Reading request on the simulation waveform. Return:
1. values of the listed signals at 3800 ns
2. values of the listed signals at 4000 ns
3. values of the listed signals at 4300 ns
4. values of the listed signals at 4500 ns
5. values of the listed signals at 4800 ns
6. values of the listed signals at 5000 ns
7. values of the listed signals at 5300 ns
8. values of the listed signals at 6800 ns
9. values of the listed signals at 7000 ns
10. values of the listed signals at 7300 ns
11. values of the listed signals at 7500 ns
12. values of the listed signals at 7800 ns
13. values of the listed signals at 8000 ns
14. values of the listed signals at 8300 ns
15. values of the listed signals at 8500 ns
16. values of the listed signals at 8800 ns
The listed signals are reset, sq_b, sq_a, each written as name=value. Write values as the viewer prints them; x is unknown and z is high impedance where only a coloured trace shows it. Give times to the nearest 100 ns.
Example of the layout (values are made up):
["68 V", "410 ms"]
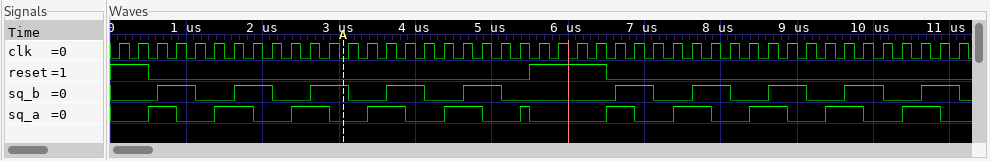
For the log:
["reset=0, sq_b=1, sq_a=1", "reset=0, sq_b=1, sq_a=0", "reset=0, sq_b=0, sq_a=0", "reset=0, sq_b=0, sq_a=1", "reset=0, sq_b=1, sq_a=1", "reset=0, sq_b=1, sq_a=0", "reset=0, sq_b=0, sq_a=0", "reset=0, sq_b=1, sq_a=1", "reset=0, sq_b=1, sq_a=0", "reset=0, sq_b=0, sq_a=0", "reset=0, sq_b=0, sq_a=1", "reset=0, sq_b=1, sq_a=1", "reset=0, sq_b=1, sq_a=0", "reset=0, sq_b=0, sq_a=0", "reset=0, sq_b=0, sq_a=1", "reset=0, sq_b=1, sq_a=1"]
